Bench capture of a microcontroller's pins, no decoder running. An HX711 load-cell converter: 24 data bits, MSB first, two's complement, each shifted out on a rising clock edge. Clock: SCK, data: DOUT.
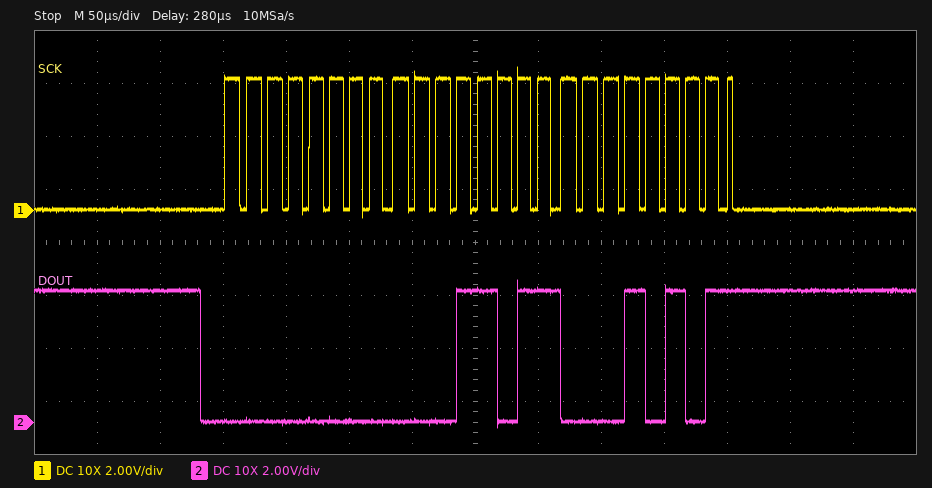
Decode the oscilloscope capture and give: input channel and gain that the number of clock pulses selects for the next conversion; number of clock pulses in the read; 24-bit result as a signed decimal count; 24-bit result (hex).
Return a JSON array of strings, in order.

["channel A, gain 128", "25", "6933", "0x001B15"]
